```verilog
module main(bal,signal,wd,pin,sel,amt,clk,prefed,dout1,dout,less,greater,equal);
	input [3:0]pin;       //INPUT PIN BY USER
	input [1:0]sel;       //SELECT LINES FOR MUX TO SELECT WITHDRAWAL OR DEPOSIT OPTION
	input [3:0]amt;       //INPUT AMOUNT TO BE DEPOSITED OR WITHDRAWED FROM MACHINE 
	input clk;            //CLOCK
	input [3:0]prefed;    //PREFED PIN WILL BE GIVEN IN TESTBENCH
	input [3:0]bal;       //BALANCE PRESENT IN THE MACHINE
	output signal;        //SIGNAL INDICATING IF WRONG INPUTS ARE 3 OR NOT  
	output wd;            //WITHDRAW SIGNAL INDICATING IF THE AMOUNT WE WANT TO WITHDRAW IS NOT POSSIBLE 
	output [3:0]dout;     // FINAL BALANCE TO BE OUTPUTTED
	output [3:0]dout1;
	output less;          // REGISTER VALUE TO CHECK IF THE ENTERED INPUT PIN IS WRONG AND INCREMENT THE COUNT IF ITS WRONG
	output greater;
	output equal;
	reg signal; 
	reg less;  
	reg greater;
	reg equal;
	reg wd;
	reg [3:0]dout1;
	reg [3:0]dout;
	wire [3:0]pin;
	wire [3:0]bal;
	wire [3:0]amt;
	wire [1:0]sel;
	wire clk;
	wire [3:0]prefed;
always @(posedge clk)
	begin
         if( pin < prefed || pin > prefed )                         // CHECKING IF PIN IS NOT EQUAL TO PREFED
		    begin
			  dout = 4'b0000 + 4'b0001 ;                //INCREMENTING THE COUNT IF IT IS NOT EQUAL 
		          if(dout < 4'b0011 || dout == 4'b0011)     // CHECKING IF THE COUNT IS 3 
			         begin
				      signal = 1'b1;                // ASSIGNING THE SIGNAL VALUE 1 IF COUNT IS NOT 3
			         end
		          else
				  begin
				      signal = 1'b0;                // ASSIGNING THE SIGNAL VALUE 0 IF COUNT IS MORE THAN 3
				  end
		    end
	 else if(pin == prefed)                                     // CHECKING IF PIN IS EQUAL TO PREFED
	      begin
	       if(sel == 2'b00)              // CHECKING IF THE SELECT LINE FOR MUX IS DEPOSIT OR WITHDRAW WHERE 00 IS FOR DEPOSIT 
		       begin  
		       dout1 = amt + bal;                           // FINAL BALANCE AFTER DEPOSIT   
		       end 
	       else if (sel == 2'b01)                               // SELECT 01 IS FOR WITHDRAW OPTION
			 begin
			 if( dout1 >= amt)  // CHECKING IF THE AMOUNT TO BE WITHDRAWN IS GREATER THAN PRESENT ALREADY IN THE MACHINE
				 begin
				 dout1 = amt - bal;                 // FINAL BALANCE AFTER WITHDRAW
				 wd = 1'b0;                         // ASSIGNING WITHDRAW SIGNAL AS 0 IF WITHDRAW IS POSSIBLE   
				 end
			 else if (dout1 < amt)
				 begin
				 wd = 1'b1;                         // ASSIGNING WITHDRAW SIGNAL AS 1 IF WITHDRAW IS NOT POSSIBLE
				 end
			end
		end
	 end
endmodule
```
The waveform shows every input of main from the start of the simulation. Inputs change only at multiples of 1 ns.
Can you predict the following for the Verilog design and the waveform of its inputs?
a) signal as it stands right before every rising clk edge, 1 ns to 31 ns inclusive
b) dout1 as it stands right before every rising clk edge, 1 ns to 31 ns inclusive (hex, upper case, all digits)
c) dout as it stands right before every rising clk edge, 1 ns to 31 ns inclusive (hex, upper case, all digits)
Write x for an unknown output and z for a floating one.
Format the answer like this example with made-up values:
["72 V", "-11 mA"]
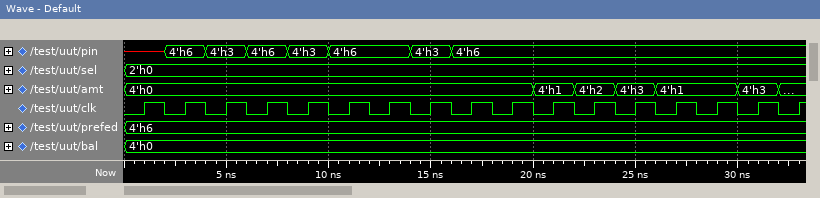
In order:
["x x x 1 1 1 1 1 1 1 1 1 1 1 1 1", "x, x, 0, 0, 0, 0, 0, 0, 0, 0, 0, 1, 2, 3, 1, 1", "x, x, x, 1, 1, 1, 1, 1, 1, 1, 1, 1, 1, 1, 1, 1"]
